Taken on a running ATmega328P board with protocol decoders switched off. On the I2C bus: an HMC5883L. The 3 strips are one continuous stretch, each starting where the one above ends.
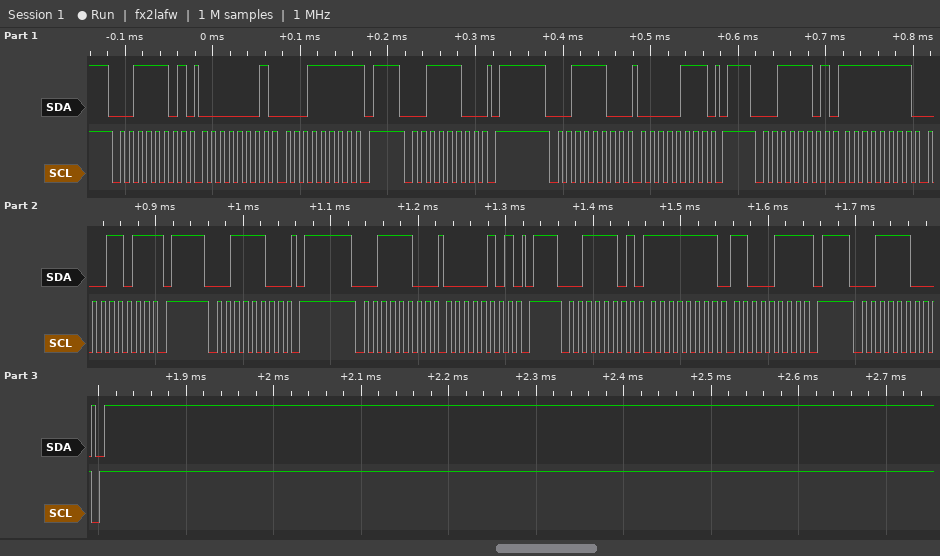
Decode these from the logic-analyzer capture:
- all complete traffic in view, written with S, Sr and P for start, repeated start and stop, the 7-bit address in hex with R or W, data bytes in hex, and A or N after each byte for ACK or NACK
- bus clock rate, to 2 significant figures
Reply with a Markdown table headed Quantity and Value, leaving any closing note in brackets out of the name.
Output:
| Quantity | Value |
|---|---|
| all complete traffic in view, written with S, Sr and P for start, repeated start and stop, the 7-bit address in hex with R or W, data bytes in hex, and A or N after each byte for ACK or NACK | S 1ER A 01 A 1F N P S 1EW A P S 1EW A 07 A P S 1ER A FF A 1B N P S 1EW A P S 1EW A 05 A P S 1ER A FF A C7 N P S 1EW A P |
| bus clock rate, to 2 significant figures | 100 kHz |
